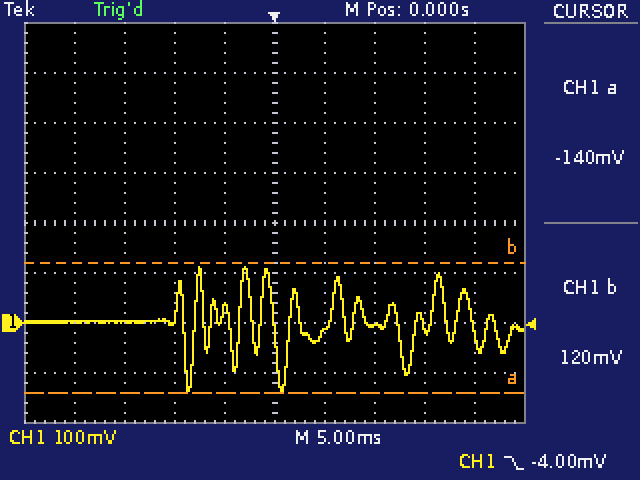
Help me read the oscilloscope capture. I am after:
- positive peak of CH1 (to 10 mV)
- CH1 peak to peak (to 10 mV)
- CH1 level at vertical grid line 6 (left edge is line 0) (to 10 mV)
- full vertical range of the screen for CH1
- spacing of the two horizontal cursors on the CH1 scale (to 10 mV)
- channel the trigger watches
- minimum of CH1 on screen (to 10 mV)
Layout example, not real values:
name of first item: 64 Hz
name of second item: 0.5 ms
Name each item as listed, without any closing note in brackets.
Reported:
positive peak of CH1: 110 mV
CH1 peak to peak: 250 mV
CH1 level at vertical grid line 6 (left edge is line 0): -20 mV
full vertical range of the screen for CH1: 800 mV
spacing of the two horizontal cursors on the CH1 scale: 260 mV
channel the trigger watches: CH1
minimum of CH1 on screen: -140 mV
